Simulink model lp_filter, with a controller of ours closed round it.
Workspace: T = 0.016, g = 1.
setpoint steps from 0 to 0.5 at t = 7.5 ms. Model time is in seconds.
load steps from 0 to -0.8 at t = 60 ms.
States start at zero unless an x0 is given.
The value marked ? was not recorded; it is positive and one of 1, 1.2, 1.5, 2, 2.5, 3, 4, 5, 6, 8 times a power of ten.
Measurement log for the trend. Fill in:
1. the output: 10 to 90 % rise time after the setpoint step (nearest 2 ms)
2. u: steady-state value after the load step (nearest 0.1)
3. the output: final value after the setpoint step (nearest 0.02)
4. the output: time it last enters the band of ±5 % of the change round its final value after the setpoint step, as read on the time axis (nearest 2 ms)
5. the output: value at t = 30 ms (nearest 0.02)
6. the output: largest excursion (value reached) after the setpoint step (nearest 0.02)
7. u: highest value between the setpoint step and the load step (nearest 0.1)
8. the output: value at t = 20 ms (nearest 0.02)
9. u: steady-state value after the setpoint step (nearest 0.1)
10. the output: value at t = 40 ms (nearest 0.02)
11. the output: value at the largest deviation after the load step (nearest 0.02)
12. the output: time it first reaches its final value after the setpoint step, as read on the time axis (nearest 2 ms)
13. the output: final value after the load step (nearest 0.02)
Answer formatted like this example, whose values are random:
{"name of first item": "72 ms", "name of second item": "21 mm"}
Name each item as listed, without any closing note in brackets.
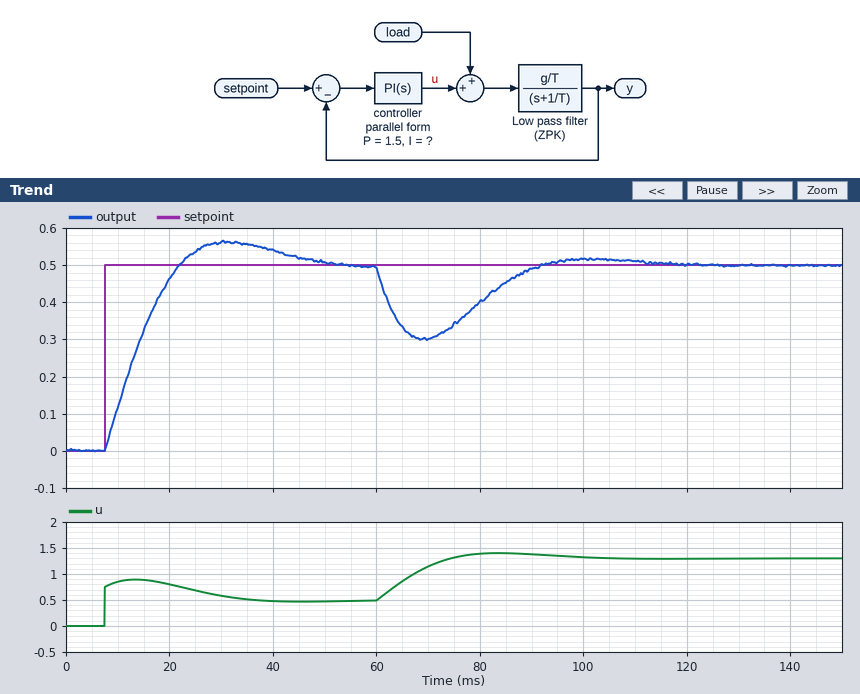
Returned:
{"the output: 10 to 90 % rise time after the setpoint step": "10 ms", "u: steady-state value after the load step": "1.3", "the output: final value after the setpoint step": "0.50", "the output: time it last enters the band of ±5 % of the change round its final value after the setpoint step, as read on the time axis": "44 ms", "the output: value at t = 30 ms": "0.56", "the output: largest excursion (value reached) after the setpoint step": "0.56", "u: highest value between the setpoint step and the load step": "0.9", "the output: value at t = 20 ms": "0.46", "u: steady-state value after the setpoint step": "0.5", "the output: value at t = 40 ms": "0.54", "the output: value at the largest deviation after the load step": "0.30", "the output: time it first reaches its final value after the setpoint step, as read on the time axis": "22 ms", "the output: final value after the load step": "0.50"}
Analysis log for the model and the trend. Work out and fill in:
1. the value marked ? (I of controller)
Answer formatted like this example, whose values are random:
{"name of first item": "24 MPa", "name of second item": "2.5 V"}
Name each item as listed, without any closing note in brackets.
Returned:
{"the value marked ?": "250"}
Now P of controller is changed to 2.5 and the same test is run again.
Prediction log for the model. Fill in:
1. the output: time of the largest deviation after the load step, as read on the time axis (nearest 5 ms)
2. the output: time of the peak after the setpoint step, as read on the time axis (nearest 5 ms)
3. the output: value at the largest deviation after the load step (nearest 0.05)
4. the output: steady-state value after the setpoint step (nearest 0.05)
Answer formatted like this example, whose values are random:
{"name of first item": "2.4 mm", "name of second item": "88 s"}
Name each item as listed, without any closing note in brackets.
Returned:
{"the output: time of the largest deviation after the load step, as read on the time axis": "70 ms", "the output: time of the peak after the setpoint step, as read on the time axis": "30 ms", "the output: value at the largest deviation after the load step": "0.35", "the output: steady-state value after the setpoint step": "0.50"}
